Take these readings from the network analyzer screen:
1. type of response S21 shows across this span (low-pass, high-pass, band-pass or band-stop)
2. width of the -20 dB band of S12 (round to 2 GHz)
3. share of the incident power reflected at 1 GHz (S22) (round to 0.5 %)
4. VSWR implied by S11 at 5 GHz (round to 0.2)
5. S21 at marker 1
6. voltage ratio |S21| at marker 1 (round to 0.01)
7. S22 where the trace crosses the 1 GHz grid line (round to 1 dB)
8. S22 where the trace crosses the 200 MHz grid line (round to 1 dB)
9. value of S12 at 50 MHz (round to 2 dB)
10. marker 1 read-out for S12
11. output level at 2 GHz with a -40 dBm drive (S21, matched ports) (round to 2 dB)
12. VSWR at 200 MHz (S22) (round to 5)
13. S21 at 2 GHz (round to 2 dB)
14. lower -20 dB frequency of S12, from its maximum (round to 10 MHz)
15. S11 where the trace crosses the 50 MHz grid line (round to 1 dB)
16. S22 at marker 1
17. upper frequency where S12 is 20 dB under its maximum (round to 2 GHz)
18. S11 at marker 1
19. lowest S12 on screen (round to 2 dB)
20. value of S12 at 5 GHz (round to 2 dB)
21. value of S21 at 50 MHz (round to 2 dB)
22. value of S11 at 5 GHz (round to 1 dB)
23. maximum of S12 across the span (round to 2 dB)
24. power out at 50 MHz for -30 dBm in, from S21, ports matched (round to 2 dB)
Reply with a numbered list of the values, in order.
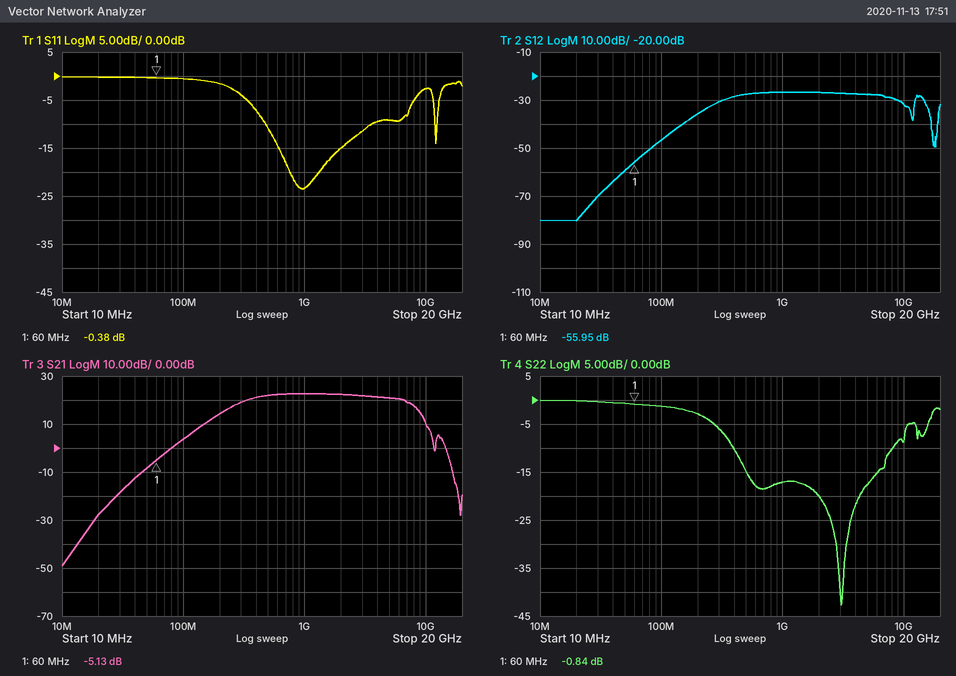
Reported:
1. band-pass
2. 18 GHz
3. 2.0 %
4. 2.0
5. -5.13 dB
6. 0.55
7. -17 dB
8. -3 dB
9. -60 dB
10. -55.95 dB
11. -18 dBm
12. 5
13. 22 dB
14. 100 MHz
15. 0 dB
16. -0.84 dB
17. 18 GHz
18. -0.38 dB
19. -80 dB
20. -28 dB
21. -8 dB
22. -9 dB
23. -26 dB
24. -38 dBm
